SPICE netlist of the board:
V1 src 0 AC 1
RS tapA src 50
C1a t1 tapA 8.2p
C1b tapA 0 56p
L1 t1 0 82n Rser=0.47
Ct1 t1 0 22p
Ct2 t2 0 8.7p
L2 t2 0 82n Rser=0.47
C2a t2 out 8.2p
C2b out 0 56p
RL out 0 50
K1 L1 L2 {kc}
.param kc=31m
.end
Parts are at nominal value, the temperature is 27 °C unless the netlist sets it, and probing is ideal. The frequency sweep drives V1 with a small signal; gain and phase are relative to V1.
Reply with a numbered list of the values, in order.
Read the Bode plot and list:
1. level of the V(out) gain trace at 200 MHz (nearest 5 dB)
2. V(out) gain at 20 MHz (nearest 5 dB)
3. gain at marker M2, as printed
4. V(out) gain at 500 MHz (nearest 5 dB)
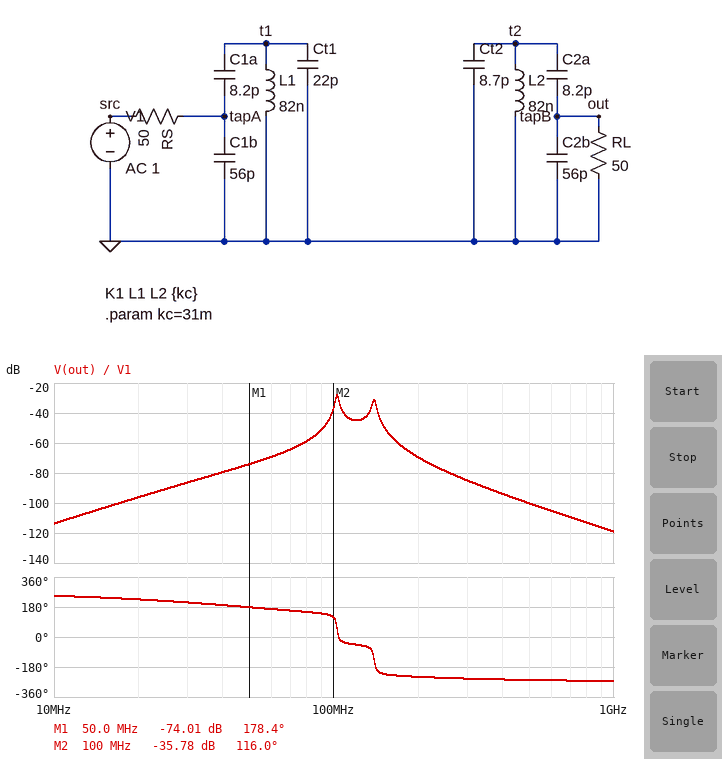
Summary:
1. -70 dB
2. -95 dB
3. -35.78 dB
4. -100 dB
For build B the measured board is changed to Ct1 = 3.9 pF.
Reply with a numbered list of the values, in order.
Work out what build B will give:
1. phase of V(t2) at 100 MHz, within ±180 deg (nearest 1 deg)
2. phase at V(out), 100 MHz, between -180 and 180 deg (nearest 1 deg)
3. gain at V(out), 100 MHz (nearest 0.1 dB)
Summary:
1. 113 deg
2. 139 deg
3. -57.3 dB
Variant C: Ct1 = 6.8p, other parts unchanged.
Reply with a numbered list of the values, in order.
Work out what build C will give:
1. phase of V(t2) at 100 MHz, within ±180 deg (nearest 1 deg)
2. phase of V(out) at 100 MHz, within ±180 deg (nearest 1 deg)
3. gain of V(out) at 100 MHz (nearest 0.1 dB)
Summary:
1. 112 deg
2. 139 deg
3. -55.9 dB
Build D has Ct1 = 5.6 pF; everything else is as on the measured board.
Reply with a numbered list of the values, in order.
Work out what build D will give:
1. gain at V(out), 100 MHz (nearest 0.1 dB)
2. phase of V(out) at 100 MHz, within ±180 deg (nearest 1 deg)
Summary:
1. -56.5 dB
2. 139 deg
